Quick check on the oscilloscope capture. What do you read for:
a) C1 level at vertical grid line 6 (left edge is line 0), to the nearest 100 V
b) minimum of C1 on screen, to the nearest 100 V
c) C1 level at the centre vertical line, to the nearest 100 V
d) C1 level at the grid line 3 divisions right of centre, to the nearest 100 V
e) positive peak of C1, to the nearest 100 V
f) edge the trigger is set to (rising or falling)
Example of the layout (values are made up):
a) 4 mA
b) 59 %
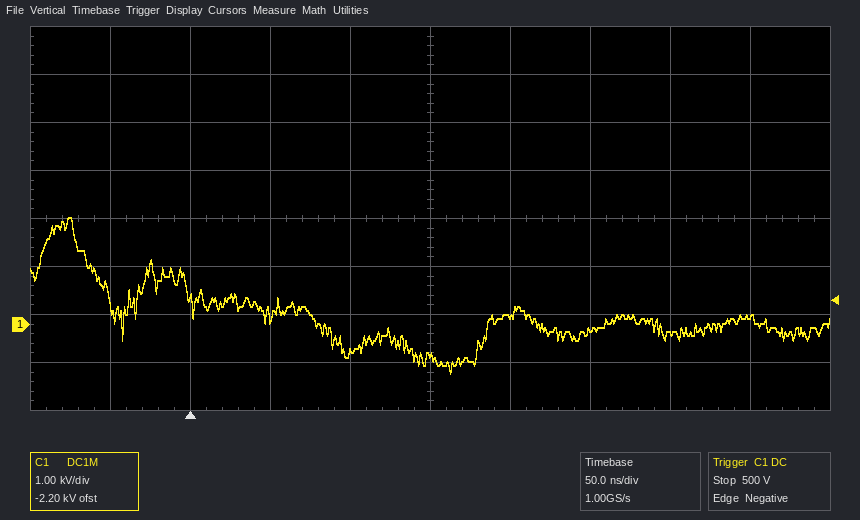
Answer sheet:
a) 200 V
b) -1.0 kV
c) -700 V
d) -200 V
e) 2.2 kV
f) falling
